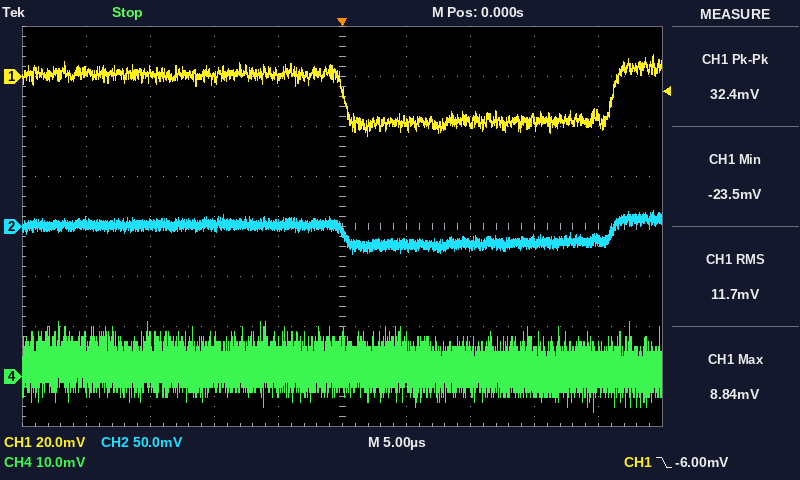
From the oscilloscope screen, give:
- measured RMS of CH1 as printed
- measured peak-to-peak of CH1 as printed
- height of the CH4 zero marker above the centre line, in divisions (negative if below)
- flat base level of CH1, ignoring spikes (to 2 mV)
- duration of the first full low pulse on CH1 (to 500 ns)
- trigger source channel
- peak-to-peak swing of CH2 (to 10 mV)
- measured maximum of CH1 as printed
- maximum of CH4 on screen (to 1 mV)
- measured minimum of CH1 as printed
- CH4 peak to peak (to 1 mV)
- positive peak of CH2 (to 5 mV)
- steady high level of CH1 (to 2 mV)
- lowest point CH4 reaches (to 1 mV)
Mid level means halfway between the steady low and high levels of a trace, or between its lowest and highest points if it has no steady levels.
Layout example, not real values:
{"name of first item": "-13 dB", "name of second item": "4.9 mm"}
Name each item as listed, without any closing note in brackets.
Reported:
{"measured RMS of CH1 as printed": "11.7 mV", "measured peak-to-peak of CH1 as printed": "32.4 mV", "height of the CH4 zero marker above the centre line, in divisions": "-3.0 div", "flat base level of CH1, ignoring spikes": "-18 mV", "duration of the first full low pulse on CH1": "21.0 µs", "trigger source channel": "CH1", "peak-to-peak swing of CH2": "40 mV", "measured maximum of CH1 as printed": "8.84 mV", "maximum of CH4 on screen": "11 mV", "measured minimum of CH1 as printed": "-23.5 mV", "CH4 peak to peak": "18 mV", "positive peak of CH2": "15 mV", "steady high level of CH1": "2 mV", "lowest point CH4 reaches": "-7 mV"}
